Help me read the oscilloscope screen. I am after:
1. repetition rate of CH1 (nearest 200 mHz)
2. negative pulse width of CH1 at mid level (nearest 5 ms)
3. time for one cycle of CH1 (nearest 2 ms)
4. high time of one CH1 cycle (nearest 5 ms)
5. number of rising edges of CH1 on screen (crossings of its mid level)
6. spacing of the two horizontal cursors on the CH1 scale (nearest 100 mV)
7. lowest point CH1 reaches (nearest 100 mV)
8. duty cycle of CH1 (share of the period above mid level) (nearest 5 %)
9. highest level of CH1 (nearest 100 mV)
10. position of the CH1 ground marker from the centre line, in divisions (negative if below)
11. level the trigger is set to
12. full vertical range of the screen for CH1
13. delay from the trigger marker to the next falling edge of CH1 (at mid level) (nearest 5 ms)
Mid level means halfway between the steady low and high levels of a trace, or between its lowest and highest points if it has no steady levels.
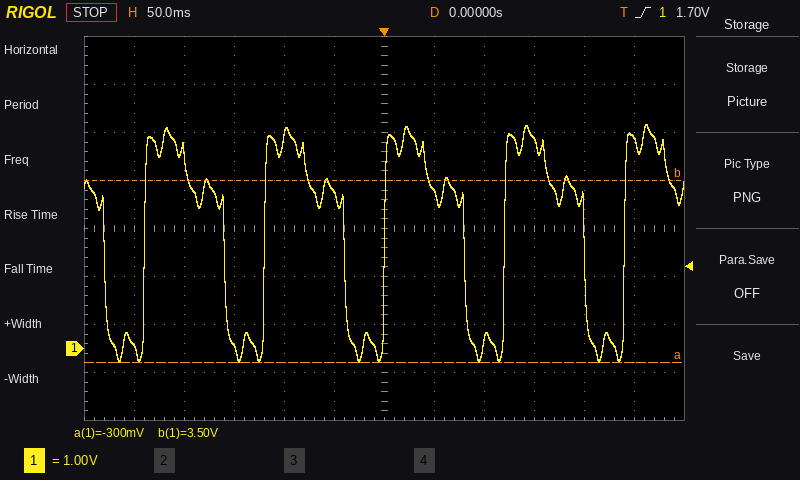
8.4 Hz
40 ms
120 ms
80 ms
5
3.8 V
-300 mV
65 %
4.7 V
-2.5 div
1.70 V
8 V
80 ms
